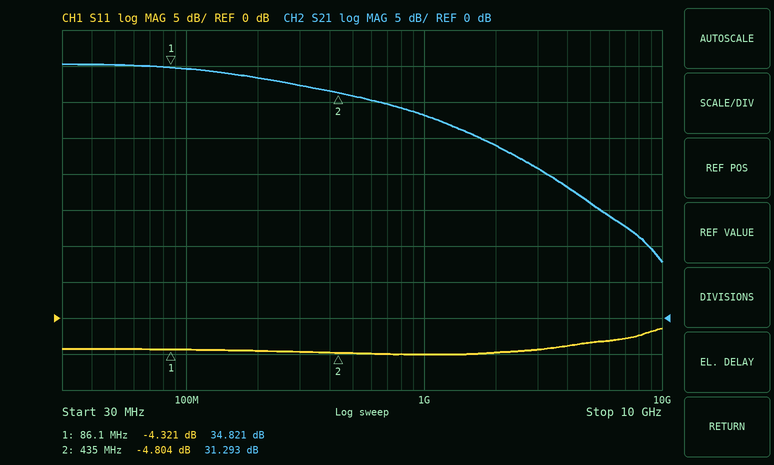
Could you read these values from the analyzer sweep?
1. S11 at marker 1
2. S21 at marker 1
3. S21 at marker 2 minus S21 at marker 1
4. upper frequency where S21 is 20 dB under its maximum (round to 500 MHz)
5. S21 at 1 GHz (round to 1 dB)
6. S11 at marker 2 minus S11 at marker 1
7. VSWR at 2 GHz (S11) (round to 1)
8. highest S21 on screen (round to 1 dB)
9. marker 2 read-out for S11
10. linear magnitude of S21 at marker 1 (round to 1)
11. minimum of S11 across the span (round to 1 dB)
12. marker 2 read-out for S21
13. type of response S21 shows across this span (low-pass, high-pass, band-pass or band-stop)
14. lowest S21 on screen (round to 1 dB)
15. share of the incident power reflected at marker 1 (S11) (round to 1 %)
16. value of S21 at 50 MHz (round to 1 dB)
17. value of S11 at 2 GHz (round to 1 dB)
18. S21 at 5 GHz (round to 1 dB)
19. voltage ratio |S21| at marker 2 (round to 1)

-4.321 dB
34.821 dB
-3.528 dB
5.5 GHz
28 dB
-0.483 dB
4
35 dB
-4.804 dB
55
-5 dB
31.293 dB
low-pass
8 dB
37 %
35 dB
-5 dB
16 dB
37
